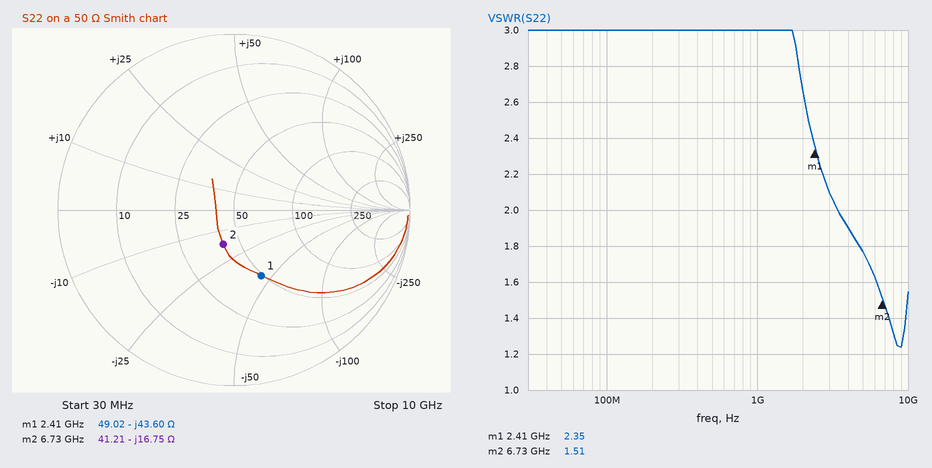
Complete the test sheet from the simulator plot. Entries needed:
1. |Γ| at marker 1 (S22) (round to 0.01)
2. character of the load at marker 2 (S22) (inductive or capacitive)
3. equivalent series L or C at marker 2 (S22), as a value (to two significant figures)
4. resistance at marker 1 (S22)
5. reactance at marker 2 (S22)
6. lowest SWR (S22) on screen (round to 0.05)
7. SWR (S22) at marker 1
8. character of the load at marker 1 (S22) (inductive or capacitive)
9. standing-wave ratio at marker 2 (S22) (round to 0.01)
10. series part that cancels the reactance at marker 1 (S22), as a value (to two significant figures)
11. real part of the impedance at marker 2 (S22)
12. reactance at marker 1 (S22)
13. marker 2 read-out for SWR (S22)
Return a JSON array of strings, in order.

["0.40", "capacitive", "1.4 pF", "49.02 Ω", "-16.75 Ω", "1.25", "2.35", "capacitive", "1.51", "2.9 nH", "41.21 Ω", "-43.60 Ω", "1.51"]
